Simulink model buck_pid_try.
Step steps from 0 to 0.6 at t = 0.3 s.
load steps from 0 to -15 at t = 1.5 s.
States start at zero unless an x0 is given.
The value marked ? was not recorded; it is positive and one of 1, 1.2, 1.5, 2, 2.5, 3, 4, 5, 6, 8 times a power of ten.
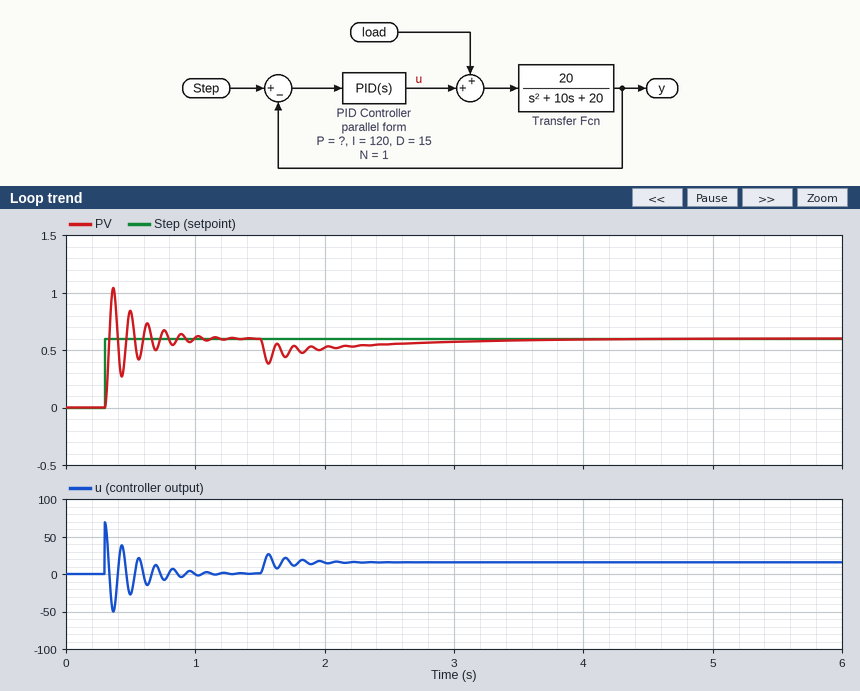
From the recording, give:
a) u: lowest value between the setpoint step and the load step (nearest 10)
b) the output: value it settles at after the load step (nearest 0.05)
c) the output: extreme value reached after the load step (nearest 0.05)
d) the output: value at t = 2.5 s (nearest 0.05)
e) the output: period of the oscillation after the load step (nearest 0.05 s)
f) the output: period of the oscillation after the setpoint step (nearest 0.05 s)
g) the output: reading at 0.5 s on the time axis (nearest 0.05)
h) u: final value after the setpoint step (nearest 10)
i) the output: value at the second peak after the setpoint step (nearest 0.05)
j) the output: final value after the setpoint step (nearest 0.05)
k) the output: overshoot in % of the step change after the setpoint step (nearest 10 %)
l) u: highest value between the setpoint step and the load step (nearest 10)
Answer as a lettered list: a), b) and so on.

a) -50
b) 0.60
c) 0.40
d) 0.55
e) 0.15 s
f) 0.15 s
g) 0.85
h) 0
i) 0.85
j) 0.60
k) 70 %
l) 70
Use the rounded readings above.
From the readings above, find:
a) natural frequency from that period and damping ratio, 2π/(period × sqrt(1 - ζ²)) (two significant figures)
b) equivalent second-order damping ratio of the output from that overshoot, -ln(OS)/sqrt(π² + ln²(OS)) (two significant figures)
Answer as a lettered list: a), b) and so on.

a) 42 rad/s
b) 0.11
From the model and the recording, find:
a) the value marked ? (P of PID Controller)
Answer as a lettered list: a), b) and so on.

a) 100
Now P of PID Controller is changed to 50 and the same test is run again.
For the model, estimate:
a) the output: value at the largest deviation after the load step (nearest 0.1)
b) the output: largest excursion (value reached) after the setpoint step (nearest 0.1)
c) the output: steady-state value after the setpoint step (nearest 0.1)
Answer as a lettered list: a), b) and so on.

a) 0.2
b) 1.0
c) 0.6
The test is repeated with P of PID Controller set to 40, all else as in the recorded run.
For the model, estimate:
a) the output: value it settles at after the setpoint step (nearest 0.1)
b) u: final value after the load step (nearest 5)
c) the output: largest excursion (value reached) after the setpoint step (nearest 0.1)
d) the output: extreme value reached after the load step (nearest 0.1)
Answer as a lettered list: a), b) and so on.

a) 0.6
b) 15
c) 1.0
d) 0.2
